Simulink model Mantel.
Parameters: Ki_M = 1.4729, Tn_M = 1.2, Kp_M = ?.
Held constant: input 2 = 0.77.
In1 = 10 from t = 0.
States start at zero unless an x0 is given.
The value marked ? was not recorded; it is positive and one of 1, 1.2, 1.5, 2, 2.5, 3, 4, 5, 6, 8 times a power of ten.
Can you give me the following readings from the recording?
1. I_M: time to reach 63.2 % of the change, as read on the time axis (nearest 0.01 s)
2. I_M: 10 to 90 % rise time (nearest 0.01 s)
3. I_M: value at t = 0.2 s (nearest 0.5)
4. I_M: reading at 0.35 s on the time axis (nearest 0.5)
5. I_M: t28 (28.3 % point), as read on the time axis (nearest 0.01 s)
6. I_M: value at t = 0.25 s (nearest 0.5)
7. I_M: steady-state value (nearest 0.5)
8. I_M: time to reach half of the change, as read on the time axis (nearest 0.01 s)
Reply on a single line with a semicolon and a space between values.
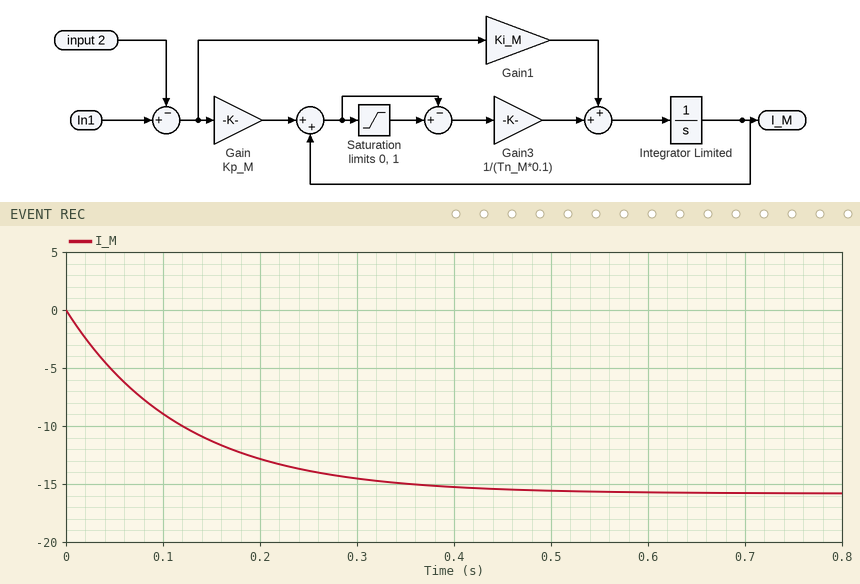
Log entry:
0.12 s; 0.26 s; -13.0; -15.0; 0.04 s; -14.0; -16.0; 0.08 s
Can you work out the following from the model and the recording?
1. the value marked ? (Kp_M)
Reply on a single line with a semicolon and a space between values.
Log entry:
2
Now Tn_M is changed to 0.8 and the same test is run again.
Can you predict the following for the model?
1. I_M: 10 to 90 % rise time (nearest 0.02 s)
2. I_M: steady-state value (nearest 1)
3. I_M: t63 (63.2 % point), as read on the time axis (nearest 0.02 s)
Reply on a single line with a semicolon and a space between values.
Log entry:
0.18 s; -16; 0.08 s
